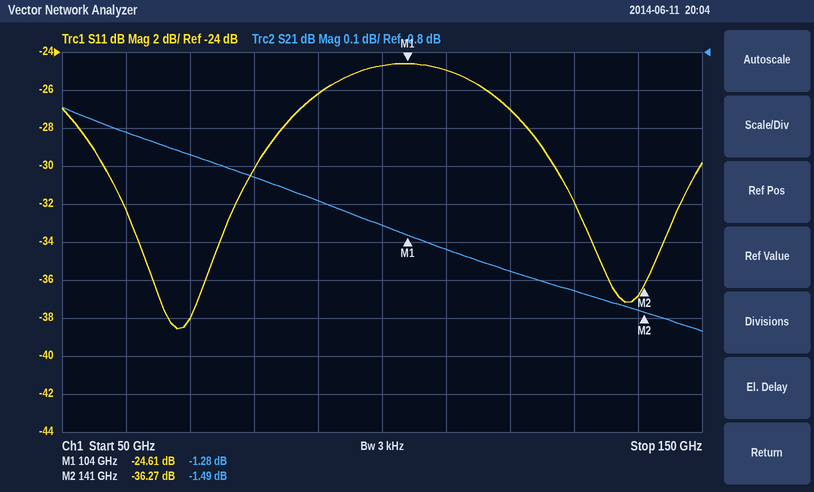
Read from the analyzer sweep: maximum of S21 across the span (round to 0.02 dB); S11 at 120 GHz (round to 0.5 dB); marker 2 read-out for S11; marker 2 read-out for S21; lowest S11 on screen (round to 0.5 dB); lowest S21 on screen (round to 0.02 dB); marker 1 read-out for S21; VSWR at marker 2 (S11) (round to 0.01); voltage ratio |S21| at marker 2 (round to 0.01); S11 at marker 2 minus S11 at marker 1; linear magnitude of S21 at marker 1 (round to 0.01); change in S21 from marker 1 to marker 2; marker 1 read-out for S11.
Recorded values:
-0.94 dB
-27.0 dB
-36.27 dB
-1.49 dB
-38.5 dB
-1.54 dB
-1.28 dB
1.03
0.84
-11.66 dB
0.86
-0.21 dB
-24.61 dB
